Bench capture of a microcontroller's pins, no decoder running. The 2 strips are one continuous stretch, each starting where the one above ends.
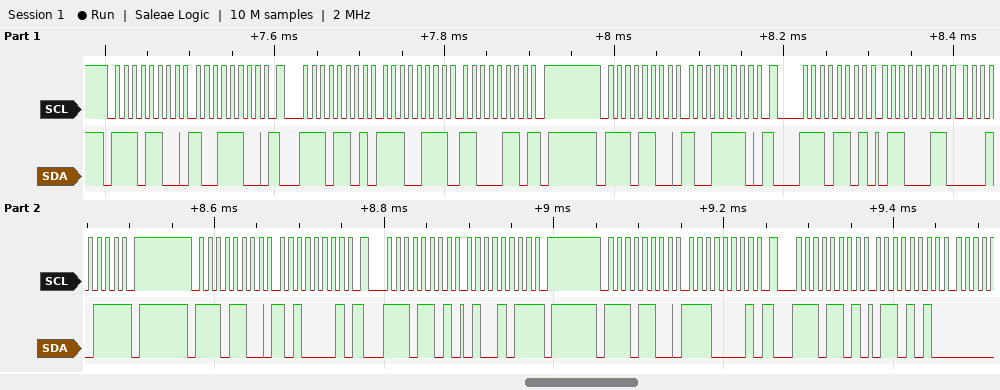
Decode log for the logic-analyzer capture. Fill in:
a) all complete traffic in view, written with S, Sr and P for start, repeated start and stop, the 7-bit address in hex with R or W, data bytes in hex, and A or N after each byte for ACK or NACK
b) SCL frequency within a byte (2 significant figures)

S 76W A 9C A Sr 76R A E7 A C6 N P S 76W A 9E A Sr 76R A 63 A 17 N P S 76W A A1 A Sr 76R A 4B N P S 76W A E1 A Sr 76R A 6A A
100 kHz
